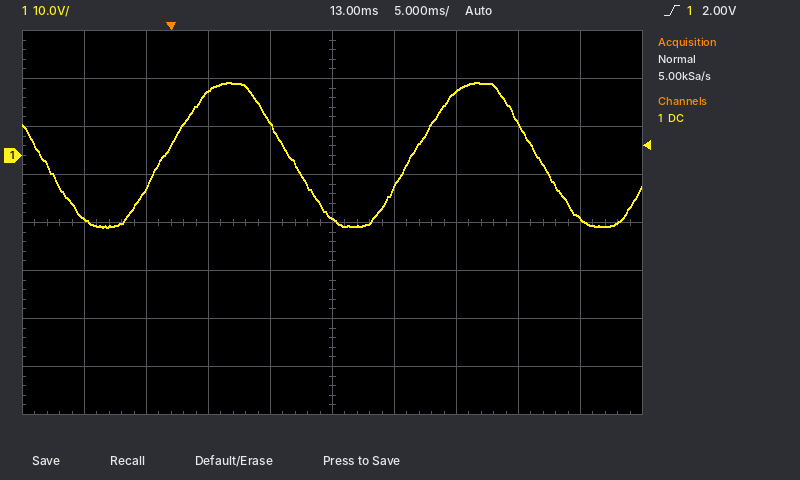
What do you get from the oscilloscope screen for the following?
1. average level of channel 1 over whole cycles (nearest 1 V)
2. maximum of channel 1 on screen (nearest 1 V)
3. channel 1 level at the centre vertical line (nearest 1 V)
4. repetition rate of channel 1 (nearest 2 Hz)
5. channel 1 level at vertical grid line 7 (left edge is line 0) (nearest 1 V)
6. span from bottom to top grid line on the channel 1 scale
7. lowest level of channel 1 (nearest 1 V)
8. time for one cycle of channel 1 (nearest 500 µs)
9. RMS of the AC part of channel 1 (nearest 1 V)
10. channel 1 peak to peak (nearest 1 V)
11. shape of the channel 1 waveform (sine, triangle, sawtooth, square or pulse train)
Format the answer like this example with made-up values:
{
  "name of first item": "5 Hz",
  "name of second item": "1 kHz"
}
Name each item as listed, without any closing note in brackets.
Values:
{
  "average level of channel 1 over whole cycles": "0 V",
  "maximum of channel 1 on screen": "15 V",
  "channel 1 level at the centre vertical line": "-13 V",
  "repetition rate of channel 1": "50 Hz",
  "channel 1 level at vertical grid line 7 (left edge is line 0)": "13 V",
  "span from bottom to top grid line on the channel 1 scale": "80 V",
  "lowest level of channel 1": "-15 V",
  "time for one cycle of channel 1": "20.0 ms",
  "RMS of the AC part of channel 1": "11 V",
  "channel 1 peak to peak": "30 V",
  "shape of the channel 1 waveform": "sine"
}
